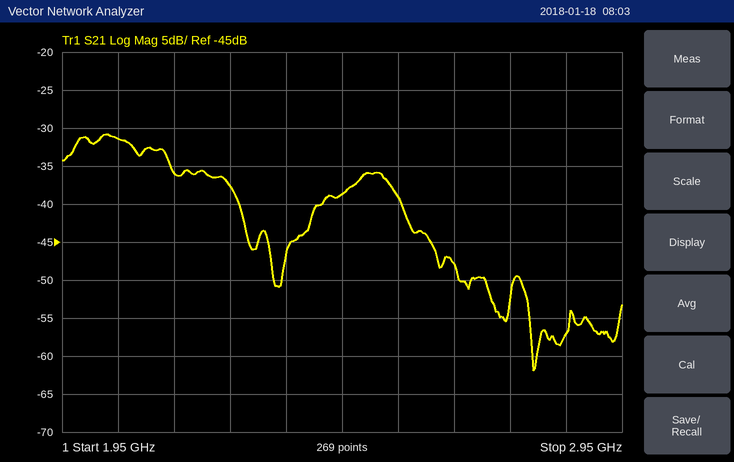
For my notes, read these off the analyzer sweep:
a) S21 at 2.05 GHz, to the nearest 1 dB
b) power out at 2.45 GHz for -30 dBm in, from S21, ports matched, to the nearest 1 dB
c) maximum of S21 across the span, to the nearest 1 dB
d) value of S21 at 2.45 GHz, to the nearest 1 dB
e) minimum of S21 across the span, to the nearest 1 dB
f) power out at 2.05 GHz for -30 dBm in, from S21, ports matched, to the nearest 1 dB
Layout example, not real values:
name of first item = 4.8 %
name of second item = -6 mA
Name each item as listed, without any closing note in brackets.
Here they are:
S21 at 2.05 GHz, to the nearest 1 dB = -31 dB
power out at 2.45 GHz for -30 dBm in, from S21, ports matched, to the nearest 1 dB = -69 dBm
maximum of S21 across the span, to the nearest 1 dB = -31 dB
value of S21 at 2.45 GHz, to the nearest 1 dB = -39 dB
minimum of S21 across the span, to the nearest 1 dB = -62 dB
power out at 2.05 GHz for -30 dBm in, from S21, ports matched, to the nearest 1 dB = -61 dBm
